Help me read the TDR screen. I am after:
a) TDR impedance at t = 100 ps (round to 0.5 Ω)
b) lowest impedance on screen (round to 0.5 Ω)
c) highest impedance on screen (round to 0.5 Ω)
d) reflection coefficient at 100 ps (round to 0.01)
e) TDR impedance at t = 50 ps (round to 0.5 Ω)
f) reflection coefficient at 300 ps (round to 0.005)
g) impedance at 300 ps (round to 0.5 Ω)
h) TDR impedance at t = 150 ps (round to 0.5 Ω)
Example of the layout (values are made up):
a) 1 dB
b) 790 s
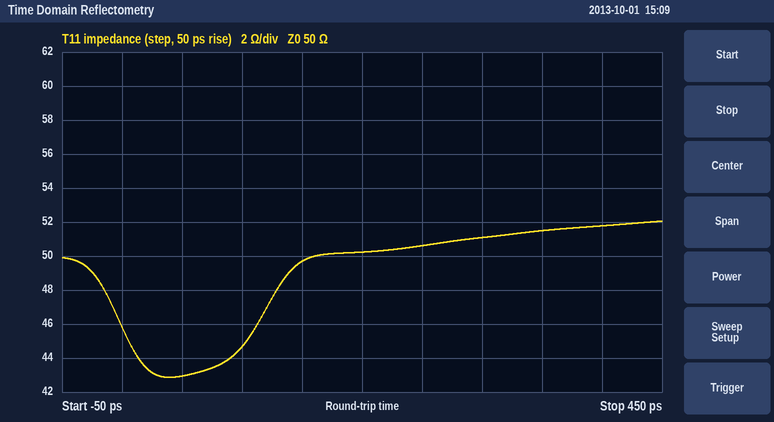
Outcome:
a) 44.5 Ω
b) 43.0 Ω
c) 52.0 Ω
d) -0.06
e) 43.0 Ω
f) +0.010
g) 51.0 Ω
h) 49.5 Ω
